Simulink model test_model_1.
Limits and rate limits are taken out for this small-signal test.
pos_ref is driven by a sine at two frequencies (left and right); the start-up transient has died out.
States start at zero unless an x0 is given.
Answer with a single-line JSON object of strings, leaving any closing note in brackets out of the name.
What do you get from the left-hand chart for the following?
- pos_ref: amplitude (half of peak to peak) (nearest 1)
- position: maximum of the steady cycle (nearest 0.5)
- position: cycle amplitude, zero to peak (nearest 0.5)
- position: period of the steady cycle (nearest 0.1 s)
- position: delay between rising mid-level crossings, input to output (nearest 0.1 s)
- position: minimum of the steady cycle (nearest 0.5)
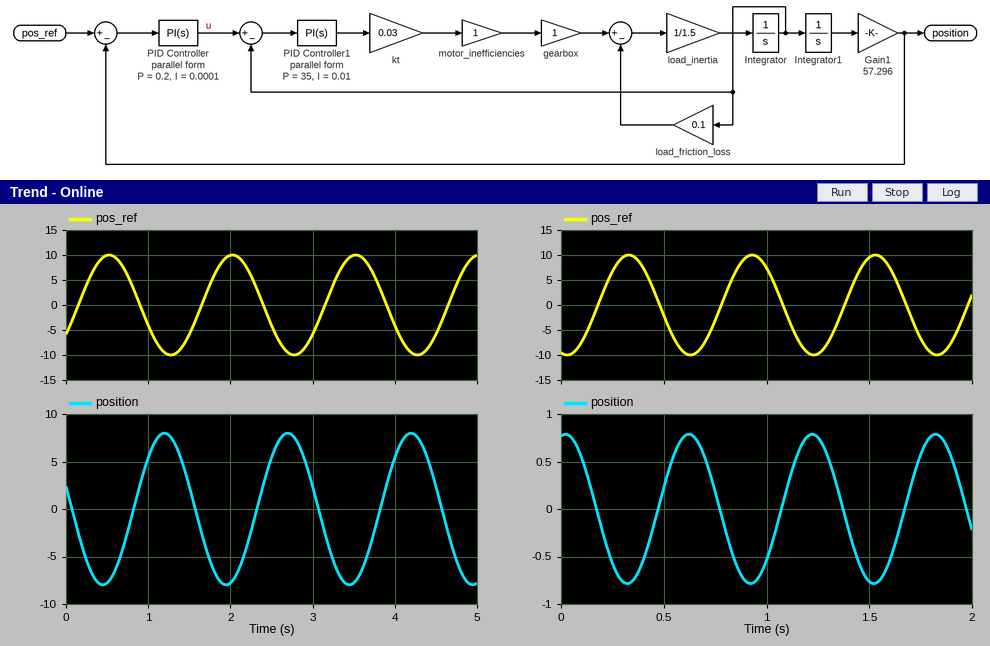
{"pos_ref: amplitude (half of peak to peak)": "10", "position: maximum of the steady cycle": "8.0", "position: cycle amplitude, zero to peak": "8.0", "position: period of the steady cycle": "1.5 s", "position: delay between rising mid-level crossings, input to output": "0.7 s", "position: minimum of the steady cycle": "-8.0"}
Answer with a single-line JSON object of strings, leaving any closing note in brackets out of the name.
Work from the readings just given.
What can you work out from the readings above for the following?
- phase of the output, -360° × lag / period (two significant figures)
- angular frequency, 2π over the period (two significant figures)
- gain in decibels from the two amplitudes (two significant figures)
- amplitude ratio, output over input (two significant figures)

{"phase of the output, -360° × lag / period": "-170°", "angular frequency, 2π over the period": "4.2 rad/s", "gain in decibels from the two amplitudes": "-1.9 dB", "amplitude ratio, output over input": "0.80"}
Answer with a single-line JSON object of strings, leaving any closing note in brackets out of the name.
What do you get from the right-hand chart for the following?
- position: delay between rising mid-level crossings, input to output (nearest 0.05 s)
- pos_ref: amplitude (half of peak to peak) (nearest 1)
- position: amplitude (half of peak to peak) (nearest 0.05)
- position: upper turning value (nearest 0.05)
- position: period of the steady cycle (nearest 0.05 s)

{"position: delay between rising mid-level crossings, input to output": "0.30 s", "pos_ref: amplitude (half of peak to peak)": "10", "position: amplitude (half of peak to peak)": "0.80", "position: upper turning value": "0.80", "position: period of the steady cycle": "0.60 s"}
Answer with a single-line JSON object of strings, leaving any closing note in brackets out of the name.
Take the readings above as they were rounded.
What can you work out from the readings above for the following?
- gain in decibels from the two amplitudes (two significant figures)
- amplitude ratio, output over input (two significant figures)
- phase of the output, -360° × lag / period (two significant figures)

{"gain in decibels from the two amplitudes": "-22 dB", "amplitude ratio, output over input": "0.080", "phase of the output, -360° × lag / period": "-180°"}
